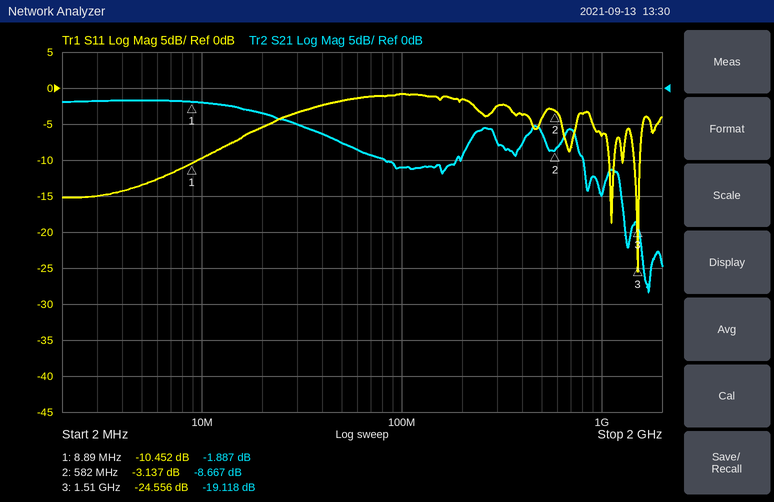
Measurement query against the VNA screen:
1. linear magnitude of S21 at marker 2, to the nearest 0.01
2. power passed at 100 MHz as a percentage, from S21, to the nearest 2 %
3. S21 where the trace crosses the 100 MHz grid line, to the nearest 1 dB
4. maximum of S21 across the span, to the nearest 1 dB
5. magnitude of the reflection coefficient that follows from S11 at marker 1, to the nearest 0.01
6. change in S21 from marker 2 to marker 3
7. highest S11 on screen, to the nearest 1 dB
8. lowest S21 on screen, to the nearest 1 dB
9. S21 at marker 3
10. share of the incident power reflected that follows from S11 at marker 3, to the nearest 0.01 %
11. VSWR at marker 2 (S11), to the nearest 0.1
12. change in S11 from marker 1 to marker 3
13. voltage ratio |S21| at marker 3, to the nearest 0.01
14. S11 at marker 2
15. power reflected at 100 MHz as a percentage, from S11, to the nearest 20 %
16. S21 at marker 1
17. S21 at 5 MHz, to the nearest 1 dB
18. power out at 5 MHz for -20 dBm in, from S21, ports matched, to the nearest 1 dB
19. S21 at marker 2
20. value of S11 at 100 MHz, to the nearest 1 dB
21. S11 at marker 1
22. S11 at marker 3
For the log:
0.37
8 %
-11 dB
-2 dB
0.30
-10.451 dB
-1 dB
-28 dB
-19.118 dB
0.35 %
5.6
-14.104 dB
0.11
-3.137 dB
80 %
-1.887 dB
-2 dB
-22 dBm
-8.667 dB
-1 dB
-10.452 dB
-24.556 dB
